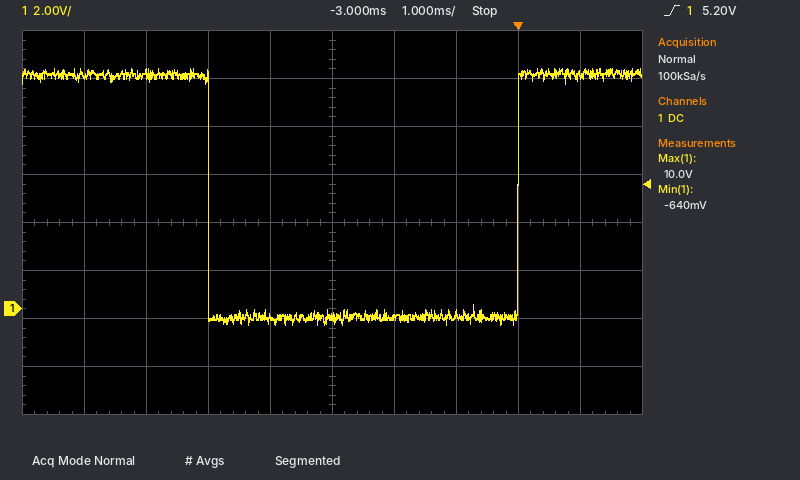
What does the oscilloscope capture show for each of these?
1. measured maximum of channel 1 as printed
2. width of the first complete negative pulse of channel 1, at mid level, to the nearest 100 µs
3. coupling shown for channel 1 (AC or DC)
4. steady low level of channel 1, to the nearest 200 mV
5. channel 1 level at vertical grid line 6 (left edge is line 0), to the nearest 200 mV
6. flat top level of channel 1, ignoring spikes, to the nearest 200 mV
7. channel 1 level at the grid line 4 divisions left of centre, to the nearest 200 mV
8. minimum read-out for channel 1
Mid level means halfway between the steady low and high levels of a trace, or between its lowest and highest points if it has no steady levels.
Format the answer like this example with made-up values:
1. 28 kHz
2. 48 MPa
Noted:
1. 10.0 V
2. 5.0 ms
3. DC
4. -400 mV
5. -400 mV
6. 9.8 V
7. 9.8 V
8. -640 mV
